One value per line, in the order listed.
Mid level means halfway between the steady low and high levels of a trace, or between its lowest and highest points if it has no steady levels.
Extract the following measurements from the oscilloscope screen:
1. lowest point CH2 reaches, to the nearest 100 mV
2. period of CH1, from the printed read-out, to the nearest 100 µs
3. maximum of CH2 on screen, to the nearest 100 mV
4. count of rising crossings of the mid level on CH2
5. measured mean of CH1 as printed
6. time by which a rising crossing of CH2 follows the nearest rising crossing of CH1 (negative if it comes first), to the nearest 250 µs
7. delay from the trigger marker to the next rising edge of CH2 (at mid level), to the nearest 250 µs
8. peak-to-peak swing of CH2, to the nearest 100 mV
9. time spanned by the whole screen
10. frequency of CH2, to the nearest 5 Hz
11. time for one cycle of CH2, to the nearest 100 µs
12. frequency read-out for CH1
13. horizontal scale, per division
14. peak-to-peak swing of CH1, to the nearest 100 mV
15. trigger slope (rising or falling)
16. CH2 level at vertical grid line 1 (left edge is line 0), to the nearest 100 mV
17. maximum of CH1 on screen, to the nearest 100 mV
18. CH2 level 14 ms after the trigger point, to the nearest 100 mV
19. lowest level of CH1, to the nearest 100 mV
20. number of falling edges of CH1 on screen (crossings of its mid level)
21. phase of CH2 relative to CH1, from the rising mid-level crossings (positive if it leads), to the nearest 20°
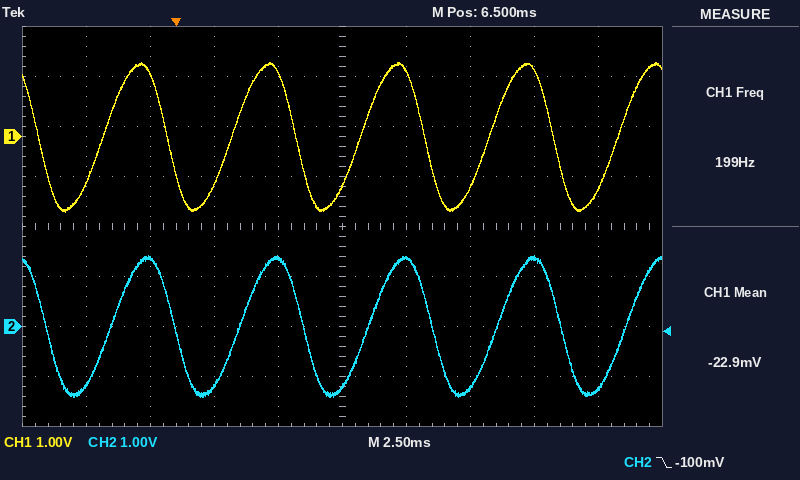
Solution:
-1.4 V
5.0 ms
1.4 V
5
-22.9 mV
+250 µs
2.50 ms
2.8 V
25 ms
200 Hz
5.0 ms
199 Hz
2.5 ms
3.0 V
falling
-1.2 V
1.5 V
1.4 V
-1.5 V
5
-20°
